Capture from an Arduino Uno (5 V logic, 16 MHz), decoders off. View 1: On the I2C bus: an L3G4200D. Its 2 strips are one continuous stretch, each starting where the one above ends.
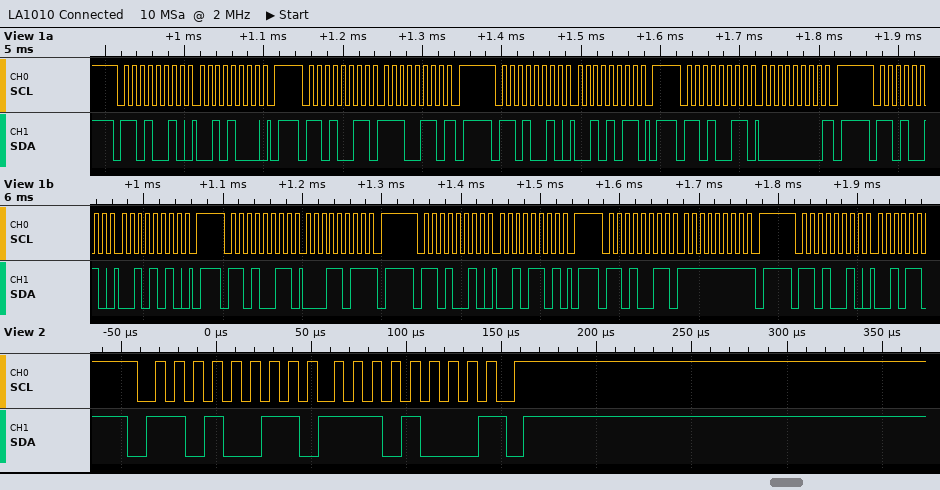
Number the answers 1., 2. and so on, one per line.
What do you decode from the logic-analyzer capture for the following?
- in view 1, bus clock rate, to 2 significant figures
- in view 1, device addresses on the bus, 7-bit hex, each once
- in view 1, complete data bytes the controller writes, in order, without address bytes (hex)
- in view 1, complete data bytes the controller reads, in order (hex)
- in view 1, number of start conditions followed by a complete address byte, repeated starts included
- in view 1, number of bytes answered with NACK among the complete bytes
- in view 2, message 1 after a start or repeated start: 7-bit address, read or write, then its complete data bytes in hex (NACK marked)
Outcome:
1. 100 kHz
2. 0x69
3. 28 2B 2A 2D
4. E6 00 1B FF
5. 9
6. 4
7. 0x69 read: E8 NACK
